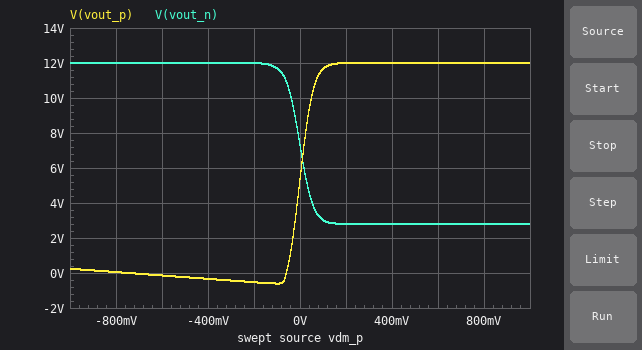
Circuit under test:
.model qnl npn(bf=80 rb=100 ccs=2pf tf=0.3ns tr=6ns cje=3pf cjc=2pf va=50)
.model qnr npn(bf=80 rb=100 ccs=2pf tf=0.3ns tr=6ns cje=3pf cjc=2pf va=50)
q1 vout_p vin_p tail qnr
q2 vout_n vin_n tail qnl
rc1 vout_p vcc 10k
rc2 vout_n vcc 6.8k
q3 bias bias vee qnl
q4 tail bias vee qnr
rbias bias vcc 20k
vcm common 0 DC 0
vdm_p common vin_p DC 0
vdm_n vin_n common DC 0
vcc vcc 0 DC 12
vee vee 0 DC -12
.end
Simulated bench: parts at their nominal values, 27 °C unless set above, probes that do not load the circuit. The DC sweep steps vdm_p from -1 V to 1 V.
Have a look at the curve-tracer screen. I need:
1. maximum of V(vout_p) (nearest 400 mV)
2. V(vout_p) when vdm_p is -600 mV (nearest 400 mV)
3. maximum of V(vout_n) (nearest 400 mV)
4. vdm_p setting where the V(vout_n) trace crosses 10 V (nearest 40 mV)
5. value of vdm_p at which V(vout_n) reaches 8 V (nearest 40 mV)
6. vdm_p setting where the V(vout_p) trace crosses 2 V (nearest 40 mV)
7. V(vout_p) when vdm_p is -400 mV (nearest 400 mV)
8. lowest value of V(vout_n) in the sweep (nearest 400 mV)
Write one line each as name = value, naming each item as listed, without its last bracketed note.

maximum of V(vout_p) = 12.0 V
V(vout_p) when vdm_p is -600 mV = 0 V
maximum of V(vout_n) = 12.0 V
vdm_p setting where the V(vout_n) trace crosses 10 V = -40 mV
value of vdm_p at which V(vout_n) reaches 8 V = 0 V
vdm_p setting where the V(vout_p) trace crosses 2 V = -40 mV
V(vout_p) when vdm_p is -400 mV = -400 mV
lowest value of V(vout_n) in the sweep = 2.8 V
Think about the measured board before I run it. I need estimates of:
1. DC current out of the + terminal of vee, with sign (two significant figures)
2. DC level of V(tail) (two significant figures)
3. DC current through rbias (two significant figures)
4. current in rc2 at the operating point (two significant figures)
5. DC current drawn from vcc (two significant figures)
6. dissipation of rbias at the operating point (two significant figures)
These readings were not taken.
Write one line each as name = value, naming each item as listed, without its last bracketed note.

DC current out of the + terminal of vee, with sign = -2.5 mA
DC level of V(tail) = -760 mV
DC current through rbias = 1.2 mA
current in rc2 at the operating point = 690 µA
DC current drawn from vcc = 2.5 mA
dissipation of rbias at the operating point = 27 mW
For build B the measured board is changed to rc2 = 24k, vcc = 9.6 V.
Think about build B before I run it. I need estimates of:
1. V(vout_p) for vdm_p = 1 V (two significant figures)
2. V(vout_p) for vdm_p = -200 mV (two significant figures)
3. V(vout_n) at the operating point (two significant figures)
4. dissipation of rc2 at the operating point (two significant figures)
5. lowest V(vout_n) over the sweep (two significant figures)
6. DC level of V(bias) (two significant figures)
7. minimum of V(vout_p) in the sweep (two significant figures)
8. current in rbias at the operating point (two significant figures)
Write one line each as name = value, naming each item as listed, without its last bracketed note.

V(vout_p) for vdm_p = 1 V = 9.6 V
V(vout_p) for vdm_p = -200 mV = -550 mV
V(vout_n) at the operating point = -710 mV
dissipation of rc2 at the operating point = 4.4 mW
lowest V(vout_n) over the sweep = -850 mV
DC level of V(bias) = -11 V
minimum of V(vout_p) in the sweep = -640 mV
current in rbias at the operating point = 1.0 mA
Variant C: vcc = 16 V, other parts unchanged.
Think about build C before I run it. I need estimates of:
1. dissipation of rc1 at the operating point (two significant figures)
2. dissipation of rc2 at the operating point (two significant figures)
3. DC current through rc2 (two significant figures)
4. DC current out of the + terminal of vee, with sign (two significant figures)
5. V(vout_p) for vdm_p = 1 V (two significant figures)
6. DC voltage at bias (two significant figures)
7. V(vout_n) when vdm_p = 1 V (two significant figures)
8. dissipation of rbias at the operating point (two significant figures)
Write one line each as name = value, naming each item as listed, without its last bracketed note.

dissipation of rc1 at the operating point = 6.1 mW
dissipation of rc2 at the operating point = 4.5 mW
DC current through rc2 = 810 µA
DC current out of the + terminal of vee, with sign = -3.0 mA
V(vout_p) for vdm_p = 1 V = 16 V
DC voltage at bias = -11 V
V(vout_n) when vdm_p = 1 V = 5.2 V
dissipation of rbias at the operating point = 37 mW
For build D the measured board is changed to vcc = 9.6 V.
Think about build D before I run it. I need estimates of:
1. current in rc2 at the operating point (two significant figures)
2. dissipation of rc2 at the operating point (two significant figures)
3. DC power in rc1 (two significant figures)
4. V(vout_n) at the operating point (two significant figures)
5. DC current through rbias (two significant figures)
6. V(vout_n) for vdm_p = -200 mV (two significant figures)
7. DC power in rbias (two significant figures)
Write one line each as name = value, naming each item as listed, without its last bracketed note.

current in rc2 at the operating point = 620 µA
dissipation of rc2 at the operating point = 2.6 mW
DC power in rc1 = 3.6 mW
V(vout_n) at the operating point = 5.4 V
DC current through rbias = 1.0 mA
V(vout_n) for vdm_p = -200 mV = 9.6 V
DC power in rbias = 22 mW
